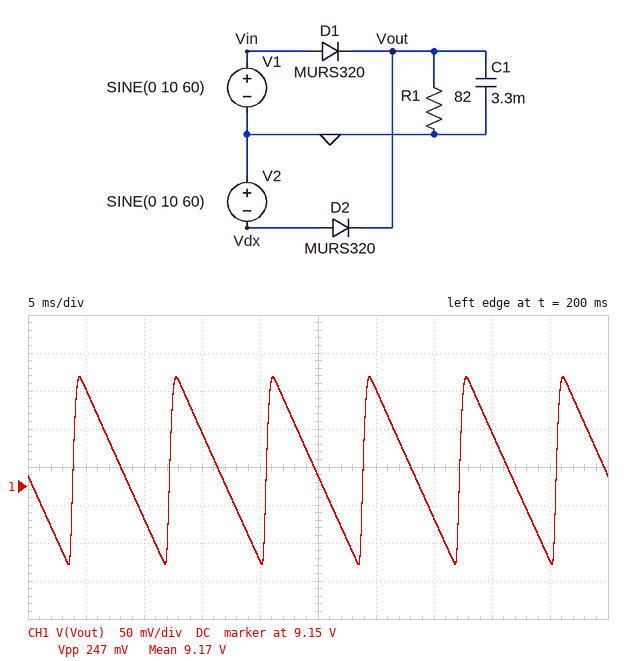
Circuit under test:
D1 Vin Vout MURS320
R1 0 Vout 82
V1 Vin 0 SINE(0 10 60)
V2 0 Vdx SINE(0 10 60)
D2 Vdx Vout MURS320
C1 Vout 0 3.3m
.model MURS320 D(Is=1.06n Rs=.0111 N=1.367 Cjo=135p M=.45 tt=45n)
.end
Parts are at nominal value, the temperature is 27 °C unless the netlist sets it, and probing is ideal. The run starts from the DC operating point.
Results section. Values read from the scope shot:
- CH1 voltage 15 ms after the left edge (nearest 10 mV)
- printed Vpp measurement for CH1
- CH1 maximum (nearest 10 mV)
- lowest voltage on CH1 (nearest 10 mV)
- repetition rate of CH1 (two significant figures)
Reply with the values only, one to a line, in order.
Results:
9.22 V
247 mV
9.29 V
9.05 V
120 Hz
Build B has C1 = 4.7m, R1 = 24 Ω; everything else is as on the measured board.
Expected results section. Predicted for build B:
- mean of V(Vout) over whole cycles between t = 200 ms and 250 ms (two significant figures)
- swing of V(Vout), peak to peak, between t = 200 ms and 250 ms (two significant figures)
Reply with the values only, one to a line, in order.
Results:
9.0 V
560 mV
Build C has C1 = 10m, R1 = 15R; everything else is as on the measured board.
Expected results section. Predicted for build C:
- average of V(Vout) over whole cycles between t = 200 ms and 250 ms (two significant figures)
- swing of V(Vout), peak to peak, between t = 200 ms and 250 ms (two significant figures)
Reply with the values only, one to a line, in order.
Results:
9.0 V
430 mV
